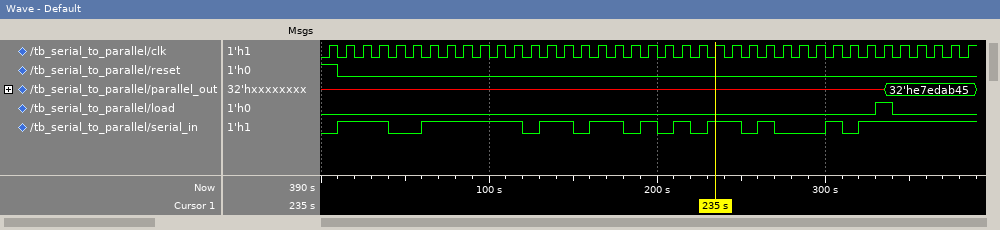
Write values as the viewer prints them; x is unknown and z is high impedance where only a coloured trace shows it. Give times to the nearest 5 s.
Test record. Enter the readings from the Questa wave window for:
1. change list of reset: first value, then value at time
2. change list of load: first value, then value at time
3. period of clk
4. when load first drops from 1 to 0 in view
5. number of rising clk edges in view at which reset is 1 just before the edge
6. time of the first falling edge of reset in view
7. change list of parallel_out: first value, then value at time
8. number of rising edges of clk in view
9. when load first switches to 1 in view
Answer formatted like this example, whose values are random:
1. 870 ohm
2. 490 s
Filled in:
1. 1, 0 at 10 s
2. 0, 1 at 330 s, 0 at 340 s
3. 10 s
4. 340 s
5. 1
6. 10 s
7. x, 32'he7edab45 at 335 s
8. 39
9. 330 s
